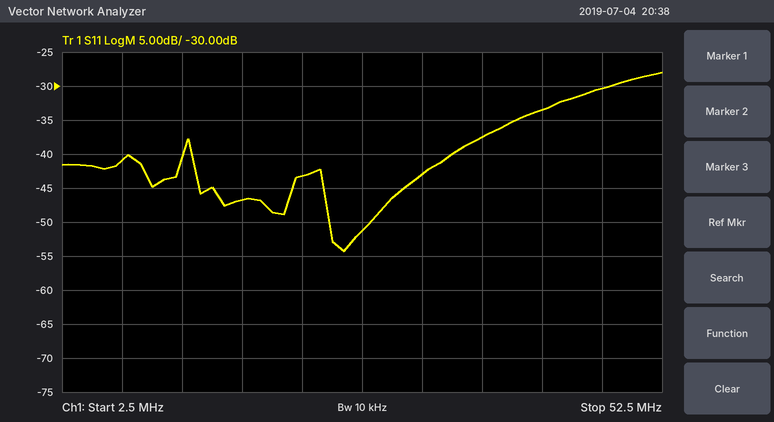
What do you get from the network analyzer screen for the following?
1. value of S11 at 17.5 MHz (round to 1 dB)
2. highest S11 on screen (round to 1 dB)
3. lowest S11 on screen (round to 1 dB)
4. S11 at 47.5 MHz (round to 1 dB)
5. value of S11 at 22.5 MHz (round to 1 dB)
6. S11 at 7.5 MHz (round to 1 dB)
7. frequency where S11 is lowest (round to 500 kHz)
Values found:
-47 dB
-28 dB
-54 dB
-30 dB
-43 dB
-41 dB
26.0 MHz
